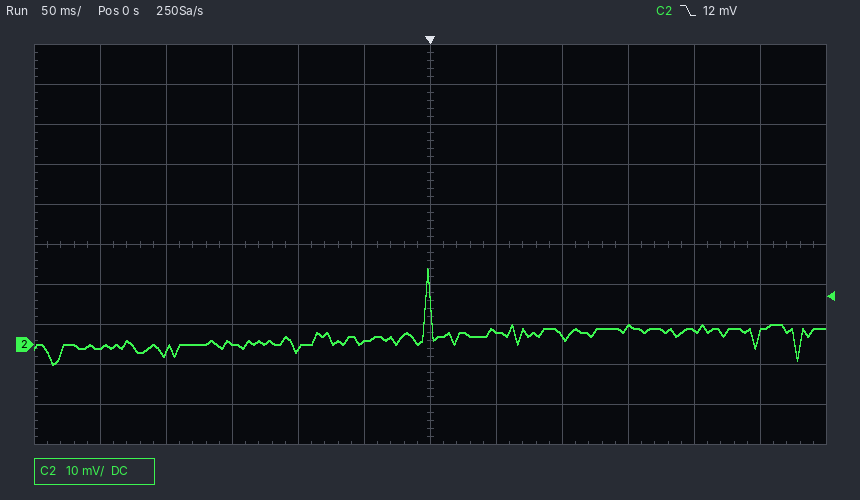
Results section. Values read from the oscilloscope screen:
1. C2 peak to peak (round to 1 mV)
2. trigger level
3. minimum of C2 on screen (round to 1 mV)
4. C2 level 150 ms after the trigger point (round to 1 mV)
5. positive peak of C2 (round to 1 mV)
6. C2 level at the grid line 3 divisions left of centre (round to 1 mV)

24 mV
12 mV
-5 mV
4 mV
19 mV
0 mV
